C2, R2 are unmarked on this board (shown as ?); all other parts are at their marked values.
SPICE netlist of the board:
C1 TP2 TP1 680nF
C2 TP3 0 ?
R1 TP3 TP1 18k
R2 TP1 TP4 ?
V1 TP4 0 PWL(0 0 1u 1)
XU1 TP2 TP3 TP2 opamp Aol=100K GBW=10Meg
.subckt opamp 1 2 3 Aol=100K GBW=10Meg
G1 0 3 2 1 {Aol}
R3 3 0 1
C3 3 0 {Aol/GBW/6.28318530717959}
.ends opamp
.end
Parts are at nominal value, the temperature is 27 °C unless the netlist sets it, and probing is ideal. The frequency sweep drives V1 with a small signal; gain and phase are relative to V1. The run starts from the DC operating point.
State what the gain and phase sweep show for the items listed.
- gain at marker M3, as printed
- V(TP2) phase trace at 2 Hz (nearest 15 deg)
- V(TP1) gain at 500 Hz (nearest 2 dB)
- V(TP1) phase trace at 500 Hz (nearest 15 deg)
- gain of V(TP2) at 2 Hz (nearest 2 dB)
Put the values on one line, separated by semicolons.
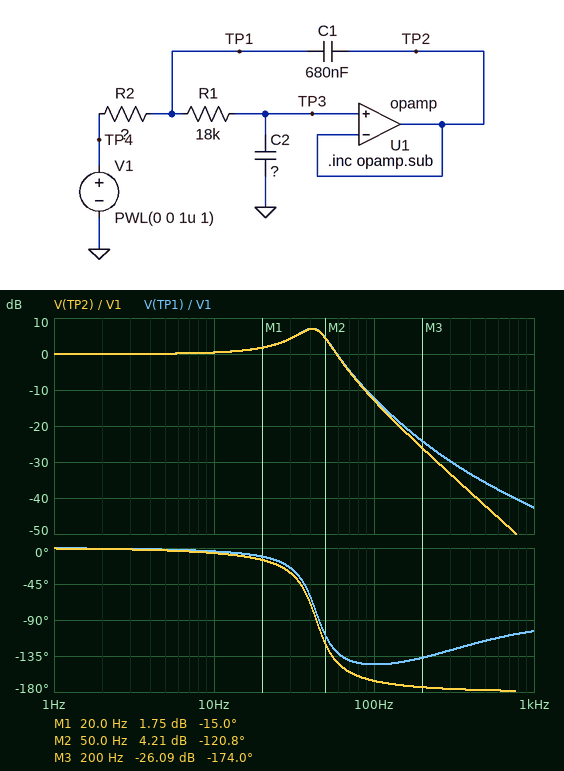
-26.09 dB; 0 deg; -36 dB; -120 deg; 0 dB
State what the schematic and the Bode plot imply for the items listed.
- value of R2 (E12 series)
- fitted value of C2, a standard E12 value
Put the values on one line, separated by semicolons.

33 kΩ; 33 nF
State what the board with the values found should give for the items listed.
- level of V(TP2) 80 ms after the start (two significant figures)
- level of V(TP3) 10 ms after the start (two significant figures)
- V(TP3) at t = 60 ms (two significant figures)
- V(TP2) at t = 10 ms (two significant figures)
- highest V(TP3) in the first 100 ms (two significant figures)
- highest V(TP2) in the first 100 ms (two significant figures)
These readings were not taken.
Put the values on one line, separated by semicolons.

1.0 V; 1.4 V; 1.0 V; 1.4 V; 1.5 V; 1.5 V
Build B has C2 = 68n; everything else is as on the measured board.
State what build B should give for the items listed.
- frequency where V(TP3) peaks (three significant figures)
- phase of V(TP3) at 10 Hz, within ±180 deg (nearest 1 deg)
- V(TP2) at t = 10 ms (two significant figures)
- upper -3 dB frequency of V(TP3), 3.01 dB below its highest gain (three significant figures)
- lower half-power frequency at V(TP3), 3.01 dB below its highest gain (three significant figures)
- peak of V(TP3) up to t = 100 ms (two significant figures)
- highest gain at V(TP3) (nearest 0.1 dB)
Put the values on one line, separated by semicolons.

26.8 Hz; -14 deg; 940 mV; 36.0 Hz; 12.0 Hz; 1.3 V; 4.1 dB
